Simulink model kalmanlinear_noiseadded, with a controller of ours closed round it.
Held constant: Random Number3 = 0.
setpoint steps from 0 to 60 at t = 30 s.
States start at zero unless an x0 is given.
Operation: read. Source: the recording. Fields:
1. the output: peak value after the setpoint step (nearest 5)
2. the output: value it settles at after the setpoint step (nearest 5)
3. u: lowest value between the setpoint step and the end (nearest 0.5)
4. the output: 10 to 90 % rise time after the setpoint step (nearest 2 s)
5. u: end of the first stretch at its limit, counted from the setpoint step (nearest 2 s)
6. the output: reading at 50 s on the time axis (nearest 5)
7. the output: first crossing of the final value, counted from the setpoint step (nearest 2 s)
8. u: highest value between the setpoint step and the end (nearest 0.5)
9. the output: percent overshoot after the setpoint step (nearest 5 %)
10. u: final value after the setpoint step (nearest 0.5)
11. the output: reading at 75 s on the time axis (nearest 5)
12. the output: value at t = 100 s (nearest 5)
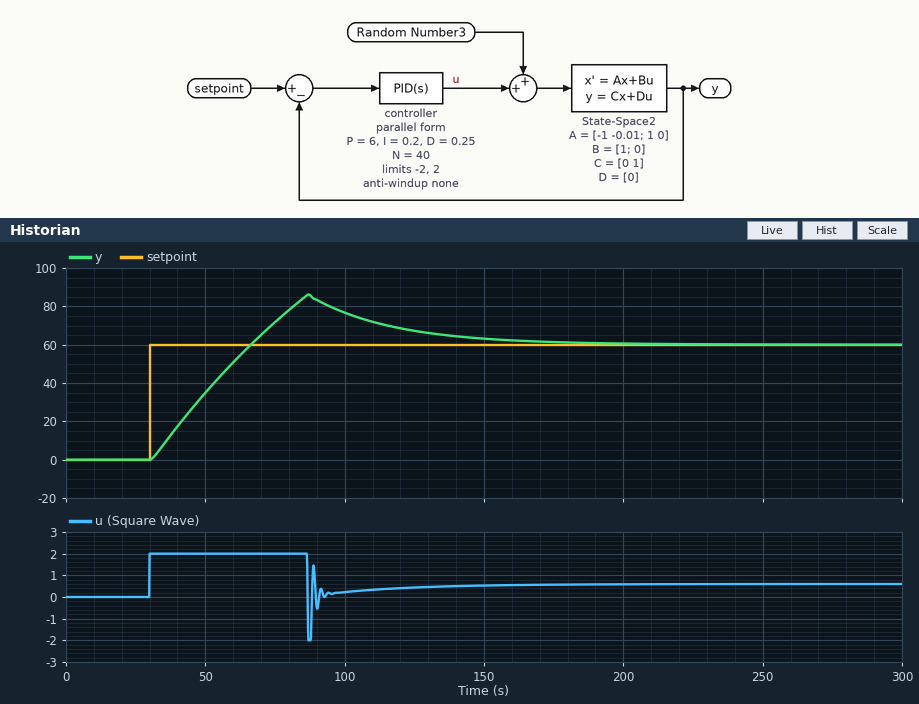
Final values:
85
60
-2.0
28 s
56 s
35
36 s
2.0
45 %
0.5
70
75
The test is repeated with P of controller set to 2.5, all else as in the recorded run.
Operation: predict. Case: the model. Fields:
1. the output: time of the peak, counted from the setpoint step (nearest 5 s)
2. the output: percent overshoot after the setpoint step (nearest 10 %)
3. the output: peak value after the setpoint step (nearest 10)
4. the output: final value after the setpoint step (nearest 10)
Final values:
65 s
60 %
100
60
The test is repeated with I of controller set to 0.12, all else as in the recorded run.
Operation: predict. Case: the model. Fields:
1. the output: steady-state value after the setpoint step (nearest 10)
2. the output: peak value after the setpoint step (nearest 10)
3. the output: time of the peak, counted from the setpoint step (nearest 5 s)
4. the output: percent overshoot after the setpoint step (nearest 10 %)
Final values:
60
80
50 s
30 %
